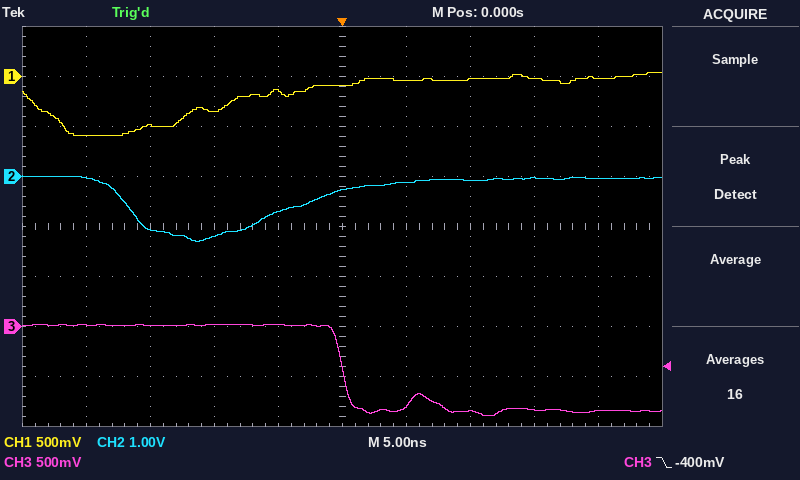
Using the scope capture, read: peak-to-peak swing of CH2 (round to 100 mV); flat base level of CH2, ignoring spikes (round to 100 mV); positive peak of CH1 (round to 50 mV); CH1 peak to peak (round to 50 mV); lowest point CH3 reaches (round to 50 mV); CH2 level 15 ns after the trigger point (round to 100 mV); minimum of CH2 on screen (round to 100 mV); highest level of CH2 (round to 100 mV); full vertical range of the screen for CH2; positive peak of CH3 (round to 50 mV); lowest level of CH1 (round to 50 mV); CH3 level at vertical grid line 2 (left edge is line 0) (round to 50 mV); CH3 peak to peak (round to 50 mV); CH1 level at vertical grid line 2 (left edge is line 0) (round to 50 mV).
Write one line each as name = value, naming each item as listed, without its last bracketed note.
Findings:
peak-to-peak swing of CH2 = 1.3 V
flat base level of CH2, ignoring spikes = -1.1 V
positive peak of CH1 = 50 mV
CH1 peak to peak = 650 mV
lowest point CH3 reaches = -900 mV
CH2 level 15 ns after the trigger point = 0.0 V
minimum of CH2 on screen = -1.3 V
highest level of CH2 = 0.0 V
full vertical range of the screen for CH2 = 8 V
positive peak of CH3 = 0 mV
lowest level of CH1 = -600 mV
CH3 level at vertical grid line 2 (left edge is line 0) = 0 mV
CH3 peak to peak = 900 mV
CH1 level at vertical grid line 2 (left edge is line 0) = -500 mV
